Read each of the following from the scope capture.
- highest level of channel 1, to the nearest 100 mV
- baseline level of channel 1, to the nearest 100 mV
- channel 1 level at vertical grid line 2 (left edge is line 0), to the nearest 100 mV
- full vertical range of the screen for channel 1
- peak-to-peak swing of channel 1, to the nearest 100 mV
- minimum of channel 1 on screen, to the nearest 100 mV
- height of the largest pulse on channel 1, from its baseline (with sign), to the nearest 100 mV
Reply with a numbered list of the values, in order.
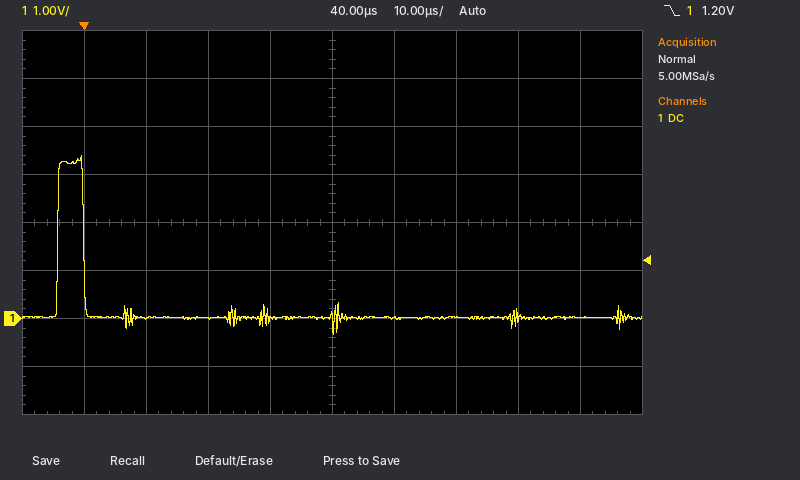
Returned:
1. 3.4 V
2. 0.0 V
3. 0.0 V
4. 8 V
5. 3.7 V
6. -300 mV
7. +3.4 V
